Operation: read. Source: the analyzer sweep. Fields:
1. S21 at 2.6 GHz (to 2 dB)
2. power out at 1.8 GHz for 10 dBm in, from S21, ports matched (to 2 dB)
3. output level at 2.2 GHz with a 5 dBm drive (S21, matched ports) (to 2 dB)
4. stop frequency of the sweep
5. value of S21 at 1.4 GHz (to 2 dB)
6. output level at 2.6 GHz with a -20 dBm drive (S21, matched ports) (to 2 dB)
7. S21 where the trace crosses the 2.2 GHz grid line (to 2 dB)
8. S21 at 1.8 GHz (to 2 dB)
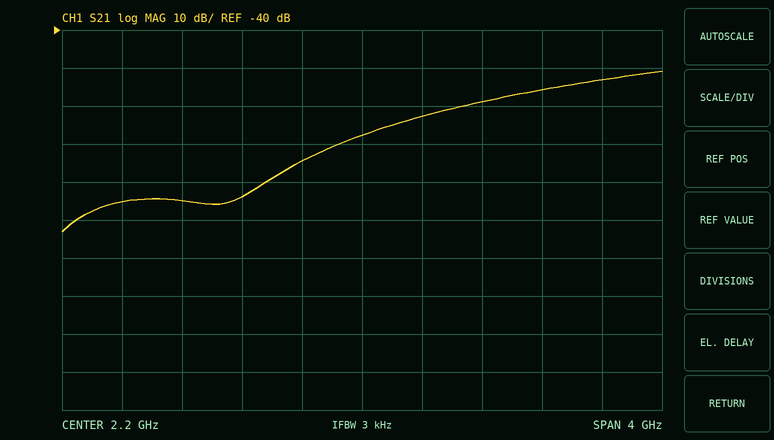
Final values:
-62 dB
-64 dBm
-62 dBm
4.2 GHz
-84 dB
-82 dBm
-68 dB
-74 dB
